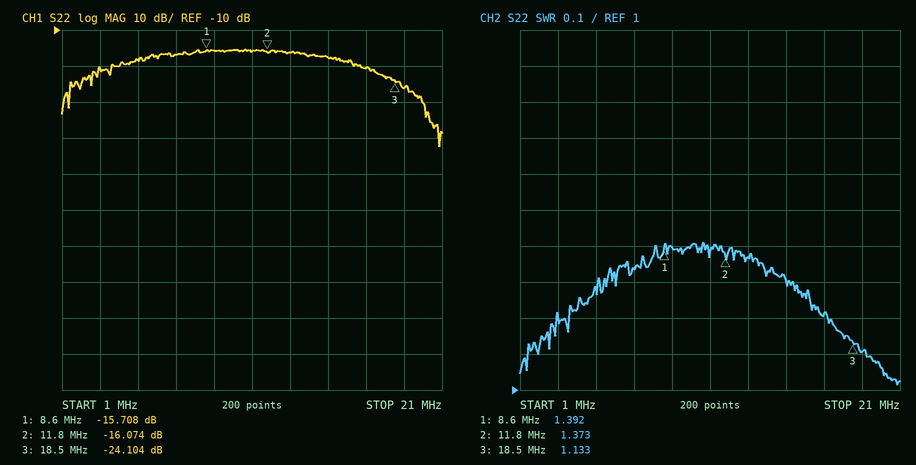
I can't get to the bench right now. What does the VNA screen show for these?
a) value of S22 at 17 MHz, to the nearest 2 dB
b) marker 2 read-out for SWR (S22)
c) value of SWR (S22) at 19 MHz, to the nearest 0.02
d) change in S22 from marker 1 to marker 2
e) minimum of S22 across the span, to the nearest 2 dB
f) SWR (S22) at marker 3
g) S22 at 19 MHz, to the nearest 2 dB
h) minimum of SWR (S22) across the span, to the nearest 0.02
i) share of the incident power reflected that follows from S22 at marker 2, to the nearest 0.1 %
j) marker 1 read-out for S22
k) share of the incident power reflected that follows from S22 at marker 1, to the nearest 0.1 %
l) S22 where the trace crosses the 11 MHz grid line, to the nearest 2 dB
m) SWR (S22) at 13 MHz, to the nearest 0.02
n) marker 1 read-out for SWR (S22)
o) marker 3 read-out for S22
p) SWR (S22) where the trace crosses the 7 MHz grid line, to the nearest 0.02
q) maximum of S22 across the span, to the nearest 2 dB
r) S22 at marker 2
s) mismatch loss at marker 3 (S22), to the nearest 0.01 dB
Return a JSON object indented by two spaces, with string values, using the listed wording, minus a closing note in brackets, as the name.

{
  "value of S22 at 17 MHz, to the nearest 2 dB": "-20 dB",
  "marker 2 read-out for SWR": "1.373",
  "value of SWR (S22) at 19 MHz, to the nearest 0.02": "1.10",
  "change in S22 from marker 1 to marker 2": "-0.366 dB",
  "minimum of S22 across the span, to the nearest 2 dB": "-42 dB",
  "SWR (S22) at marker 3": "1.133",
  "S22 at 19 MHz, to the nearest 2 dB": "-26 dB",
  "minimum of SWR (S22) across the span, to the nearest 0.02": "1.02",
  "share of the incident power reflected that follows from S22 at marker 2, to the nearest 0.1 %": "2.5 %",
  "marker 1 read-out for S22": "-15.708 dB",
  "share of the incident power reflected that follows from S22 at marker 1, to the nearest 0.1 %": "2.7 %",
  "S22 where the trace crosses the 11 MHz grid line, to the nearest 2 dB": "-16 dB",
  "SWR (S22) at 13 MHz, to the nearest 0.02": "1.36",
  "marker 1 read-out for SWR": "1.392",
  "marker 3 read-out for S22": "-24.104 dB",
  "SWR (S22) where the trace crosses the 7 MHz grid line, to the nearest 0.02": "1.34",
  "maximum of S22 across the span, to the nearest 2 dB": "-16 dB",
  "S22 at marker 2": "-16.074 dB",
  "mismatch loss at marker 3 (S22), to the nearest 0.01 dB": "0.02 dB"
}
